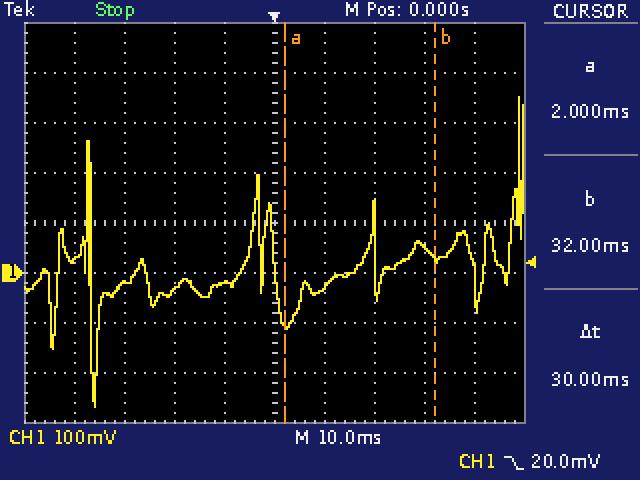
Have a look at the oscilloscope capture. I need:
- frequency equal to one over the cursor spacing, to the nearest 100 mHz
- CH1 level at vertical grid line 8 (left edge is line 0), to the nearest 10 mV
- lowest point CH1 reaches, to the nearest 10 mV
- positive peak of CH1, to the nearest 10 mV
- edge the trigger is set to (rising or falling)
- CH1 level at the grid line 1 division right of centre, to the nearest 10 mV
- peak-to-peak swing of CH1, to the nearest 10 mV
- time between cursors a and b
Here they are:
33.3 Hz
50 mV
-270 mV
350 mV
falling
-30 mV
620 mV
30 ms
